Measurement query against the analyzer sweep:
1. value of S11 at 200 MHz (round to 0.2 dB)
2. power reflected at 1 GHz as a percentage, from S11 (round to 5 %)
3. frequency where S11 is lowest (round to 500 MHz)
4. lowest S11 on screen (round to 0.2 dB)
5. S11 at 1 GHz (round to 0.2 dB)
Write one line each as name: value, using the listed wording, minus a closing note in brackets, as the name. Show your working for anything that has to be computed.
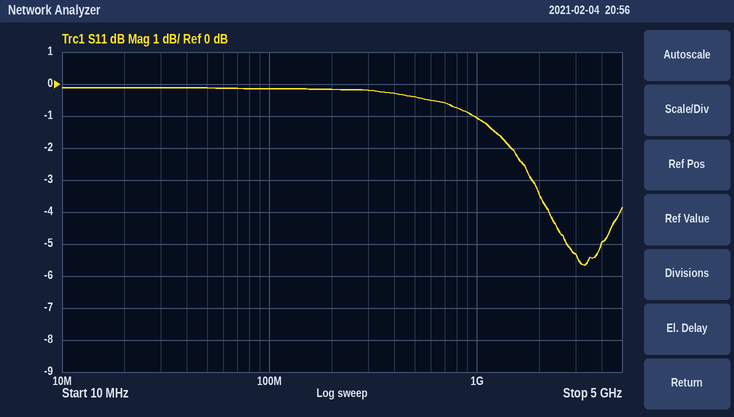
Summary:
value of S11 at 200 MHz: -0.2 dB
power reflected at 1 GHz as a percentage, from S11: 10^(-1/10) ≈ 79.4 %, so 80 % to the nearest 5 %
frequency where S11 is lowest: 3.5 GHz
lowest S11 on screen: -5.6 dB
S11 at 1 GHz: -1.0 dB
